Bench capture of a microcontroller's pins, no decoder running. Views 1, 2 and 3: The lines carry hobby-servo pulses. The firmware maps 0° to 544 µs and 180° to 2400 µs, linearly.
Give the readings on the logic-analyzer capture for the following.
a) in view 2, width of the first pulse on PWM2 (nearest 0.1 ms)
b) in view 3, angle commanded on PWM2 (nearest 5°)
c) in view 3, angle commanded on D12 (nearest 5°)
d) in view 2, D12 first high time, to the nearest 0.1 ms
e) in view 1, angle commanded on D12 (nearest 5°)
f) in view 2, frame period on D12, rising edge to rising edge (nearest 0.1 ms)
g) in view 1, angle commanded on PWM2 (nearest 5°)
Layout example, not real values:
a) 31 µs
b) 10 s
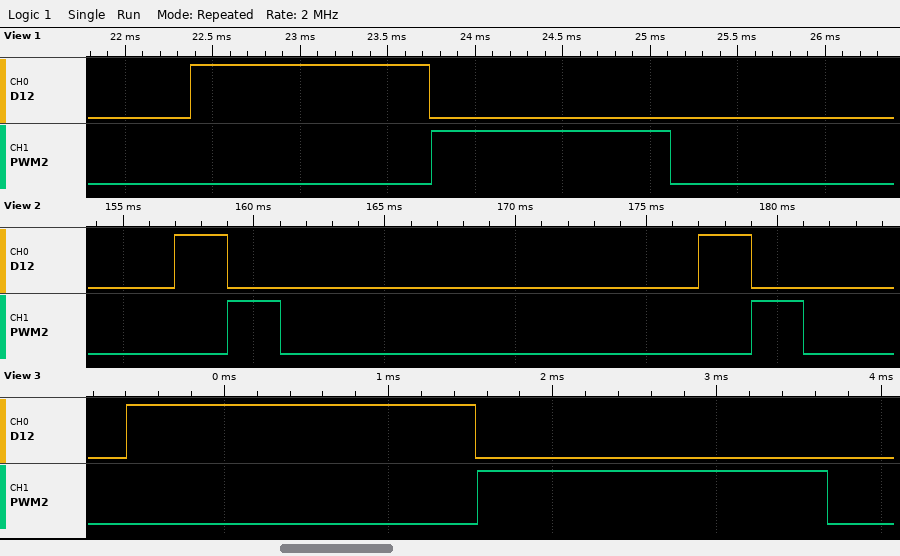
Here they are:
a) 2.0 ms
b) 155°
c) 155°
d) 2.0 ms
e) 80°
f) 20.0 ms
g) 80°
